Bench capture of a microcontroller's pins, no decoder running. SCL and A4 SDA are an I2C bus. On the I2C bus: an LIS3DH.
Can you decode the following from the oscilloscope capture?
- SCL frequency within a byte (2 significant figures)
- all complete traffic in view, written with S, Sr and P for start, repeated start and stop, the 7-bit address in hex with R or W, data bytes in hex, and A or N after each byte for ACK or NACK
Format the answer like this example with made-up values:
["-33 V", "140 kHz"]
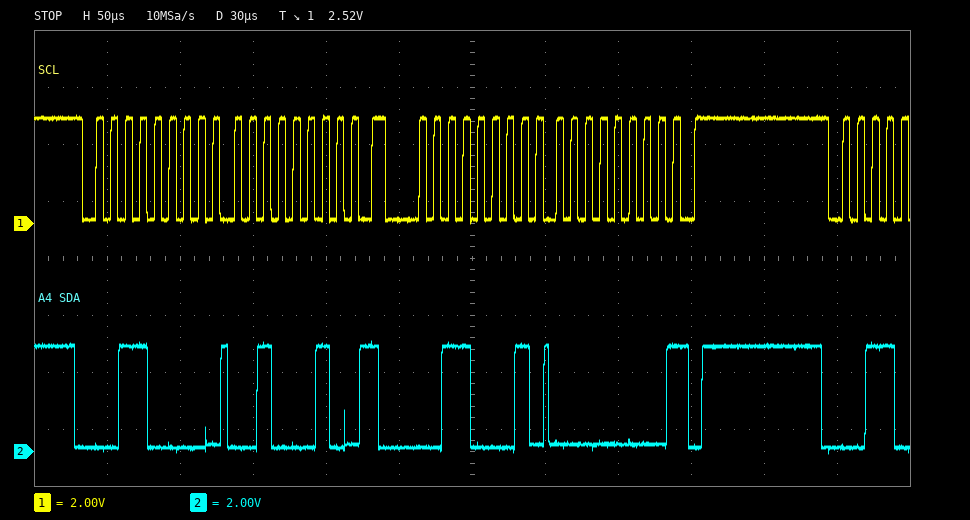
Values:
["100 kHz", "S 18W A 22 A Sr 18R A 00 N P"]
